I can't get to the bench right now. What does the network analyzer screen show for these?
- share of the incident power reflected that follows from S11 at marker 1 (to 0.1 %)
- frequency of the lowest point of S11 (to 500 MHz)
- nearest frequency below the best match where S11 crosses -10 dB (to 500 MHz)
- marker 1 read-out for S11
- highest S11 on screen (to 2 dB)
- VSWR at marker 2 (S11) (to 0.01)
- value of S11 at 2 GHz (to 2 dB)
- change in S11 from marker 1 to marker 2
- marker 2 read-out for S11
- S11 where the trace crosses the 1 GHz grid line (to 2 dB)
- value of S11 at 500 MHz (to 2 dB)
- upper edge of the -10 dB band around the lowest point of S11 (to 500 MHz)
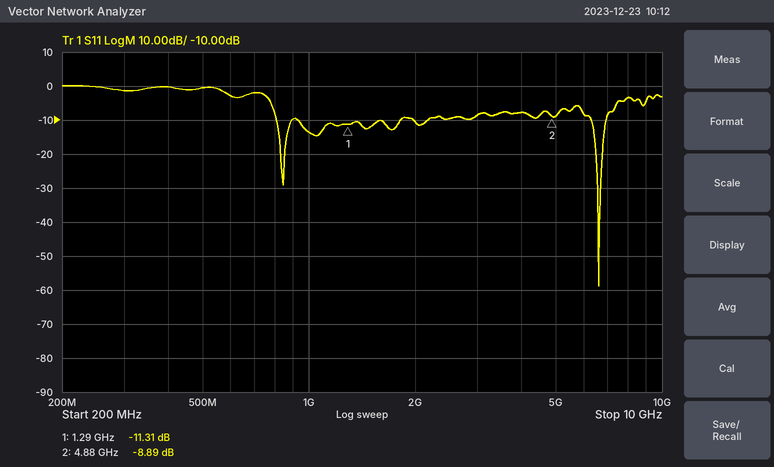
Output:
7.4 %
6.5 GHz
6.5 GHz
-11.31 dB
0 dB
2.12
-10 dB
2.42 dB
-8.89 dB
-14 dB
0 dB
7.0 GHz
